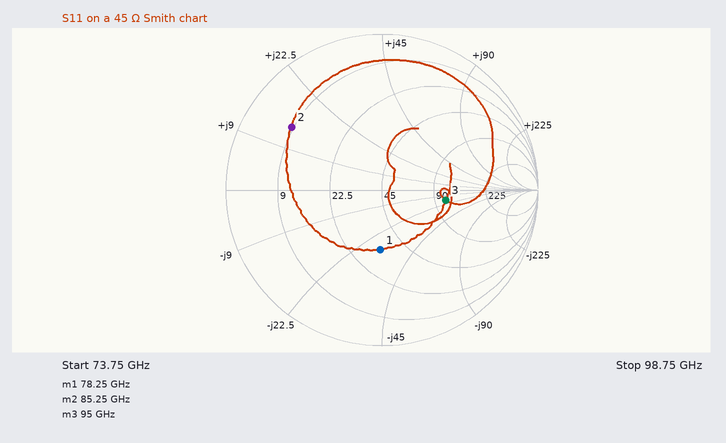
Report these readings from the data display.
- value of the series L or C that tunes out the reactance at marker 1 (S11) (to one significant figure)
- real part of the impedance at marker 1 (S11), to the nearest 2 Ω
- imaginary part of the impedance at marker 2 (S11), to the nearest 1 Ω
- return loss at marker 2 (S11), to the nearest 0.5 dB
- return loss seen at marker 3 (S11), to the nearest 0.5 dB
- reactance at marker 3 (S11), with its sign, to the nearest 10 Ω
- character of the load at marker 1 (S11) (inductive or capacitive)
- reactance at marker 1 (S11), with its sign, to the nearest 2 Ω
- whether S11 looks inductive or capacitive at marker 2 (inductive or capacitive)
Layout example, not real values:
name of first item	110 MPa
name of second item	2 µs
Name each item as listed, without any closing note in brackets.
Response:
value of the series L or C that tunes out the reactance at marker 1 (S11)	60 pH
real part of the impedance at marker 1 (S11), to the nearest 2 Ω	32 Ω
imaginary part of the impedance at marker 2 (S11), to the nearest 1 Ω	+14 Ω
return loss at marker 2 (S11), to the nearest 0.5 dB	3.0 dB
return loss seen at marker 3 (S11), to the nearest 0.5 dB	7.5 dB
reactance at marker 3 (S11), with its sign, to the nearest 10 Ω	-20 Ω
character of the load at marker 1 (S11)	capacitive
reactance at marker 1 (S11), with its sign, to the nearest 2 Ω	-30 Ω
whether S11 looks inductive or capacitive at marker 2	inductive
